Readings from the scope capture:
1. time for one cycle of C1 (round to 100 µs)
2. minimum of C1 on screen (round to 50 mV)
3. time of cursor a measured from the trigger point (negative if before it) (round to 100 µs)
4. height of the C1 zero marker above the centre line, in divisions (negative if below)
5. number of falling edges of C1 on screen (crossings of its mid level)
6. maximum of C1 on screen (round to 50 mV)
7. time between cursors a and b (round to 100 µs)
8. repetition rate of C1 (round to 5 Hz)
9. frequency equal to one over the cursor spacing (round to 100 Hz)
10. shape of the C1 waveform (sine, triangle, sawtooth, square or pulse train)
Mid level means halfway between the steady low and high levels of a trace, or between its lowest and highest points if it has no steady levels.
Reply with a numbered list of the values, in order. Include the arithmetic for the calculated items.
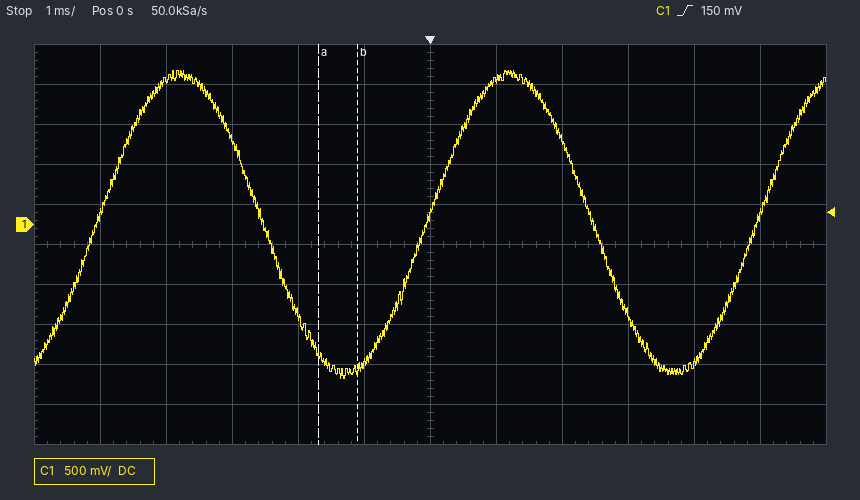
1. 5.0 ms
2. -1.90 V
3. -1.7 ms
4. +0.5 div
5. 2
6. 1.90 V
7. 600 µs
8. 1 / 5.0 ms ≈ 200 Hz
9. 1 / 600 µs ≈ 1.7 kHz
10. sine
